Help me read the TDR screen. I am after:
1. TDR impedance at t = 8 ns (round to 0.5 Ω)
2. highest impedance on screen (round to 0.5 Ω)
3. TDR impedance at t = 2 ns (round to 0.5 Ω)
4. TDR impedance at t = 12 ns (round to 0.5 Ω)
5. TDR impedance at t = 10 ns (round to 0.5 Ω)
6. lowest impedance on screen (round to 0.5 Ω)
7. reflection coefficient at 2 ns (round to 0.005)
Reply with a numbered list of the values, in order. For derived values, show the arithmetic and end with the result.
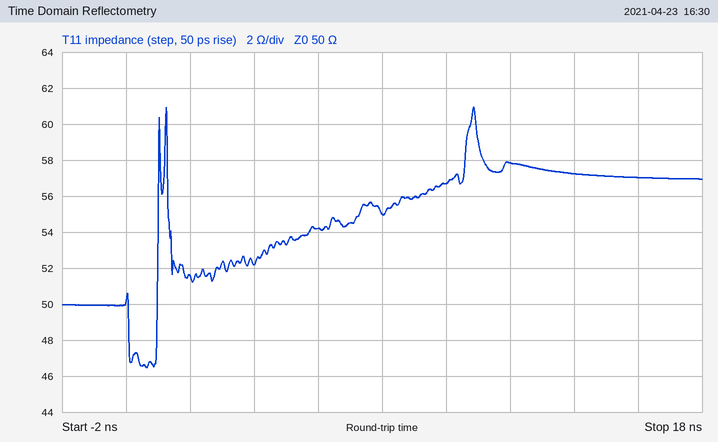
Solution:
1. 55.0 Ω
2. 61.0 Ω
3. 51.5 Ω
4. 58.0 Ω
5. 56.5 Ω
6. 46.5 Ω
7. (51.5 − 50)/(51.5 + 50) ≈ +0.015
